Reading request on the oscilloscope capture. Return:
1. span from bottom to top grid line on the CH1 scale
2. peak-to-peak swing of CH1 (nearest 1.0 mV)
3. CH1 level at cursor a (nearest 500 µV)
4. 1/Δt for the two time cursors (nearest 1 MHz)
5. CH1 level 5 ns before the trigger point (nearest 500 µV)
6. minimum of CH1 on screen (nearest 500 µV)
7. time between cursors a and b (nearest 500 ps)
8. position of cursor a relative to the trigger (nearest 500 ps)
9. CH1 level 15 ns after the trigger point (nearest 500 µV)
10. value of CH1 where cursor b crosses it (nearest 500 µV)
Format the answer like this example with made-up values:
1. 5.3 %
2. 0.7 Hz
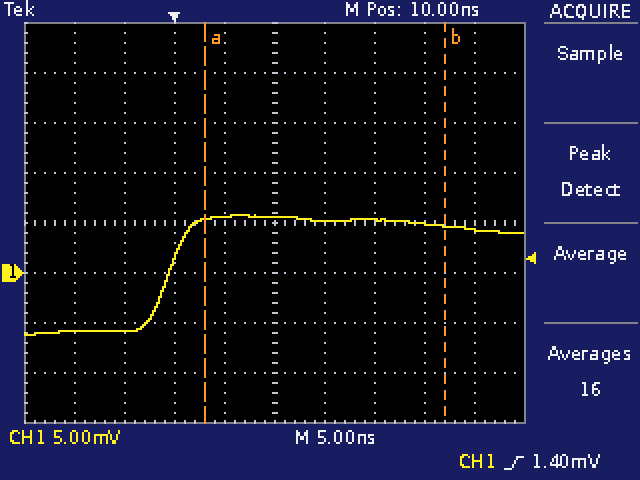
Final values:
1. 40 mV
2. 12.0 mV
3. 5.5 mV
4. 42 MHz
5. -6.0 mV
6. -6.0 mV
7. 24.0 ns
8. +3.0 ns
9. 5.0 mV
10. 4.5 mV
